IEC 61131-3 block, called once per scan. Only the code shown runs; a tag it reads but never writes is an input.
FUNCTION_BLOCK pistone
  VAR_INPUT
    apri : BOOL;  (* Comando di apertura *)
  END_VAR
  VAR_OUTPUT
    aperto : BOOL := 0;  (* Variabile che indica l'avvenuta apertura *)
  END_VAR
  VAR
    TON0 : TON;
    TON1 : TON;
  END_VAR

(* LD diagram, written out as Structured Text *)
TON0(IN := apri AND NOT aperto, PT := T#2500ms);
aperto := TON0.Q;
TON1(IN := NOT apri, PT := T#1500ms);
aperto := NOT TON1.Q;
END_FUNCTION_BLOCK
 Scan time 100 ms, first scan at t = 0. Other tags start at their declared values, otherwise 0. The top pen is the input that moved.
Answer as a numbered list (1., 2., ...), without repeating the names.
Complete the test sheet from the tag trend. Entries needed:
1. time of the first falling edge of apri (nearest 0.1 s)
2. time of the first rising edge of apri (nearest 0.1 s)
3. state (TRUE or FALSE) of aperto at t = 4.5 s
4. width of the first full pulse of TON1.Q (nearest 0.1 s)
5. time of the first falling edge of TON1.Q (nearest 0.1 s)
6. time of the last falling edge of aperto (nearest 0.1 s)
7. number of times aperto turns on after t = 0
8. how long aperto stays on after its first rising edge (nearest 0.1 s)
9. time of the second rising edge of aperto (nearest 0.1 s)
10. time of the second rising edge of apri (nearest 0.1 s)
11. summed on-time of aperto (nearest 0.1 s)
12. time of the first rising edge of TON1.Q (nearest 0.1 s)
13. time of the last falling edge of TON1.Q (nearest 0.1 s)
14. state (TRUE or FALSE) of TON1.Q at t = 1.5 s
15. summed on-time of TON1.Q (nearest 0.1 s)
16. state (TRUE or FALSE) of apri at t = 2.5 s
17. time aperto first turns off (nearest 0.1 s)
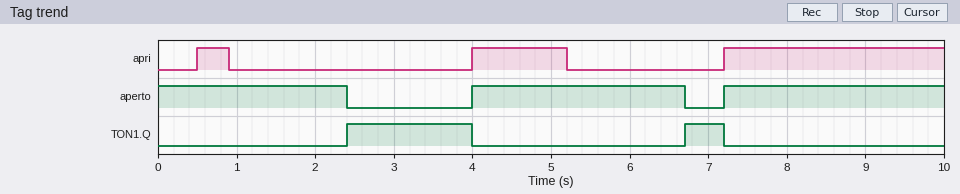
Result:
1. 0.9 s
2. 0.5 s
3. TRUE
4. 1.6 s
5. 4.0 s
6. 6.7 s
7. 2
8. 2.7 s
9. 7.2 s
10. 4.0 s
11. 7.9 s
12. 2.4 s
13. 7.2 s
14. FALSE
15. 2.1 s
16. FALSE
17. 2.4 s
